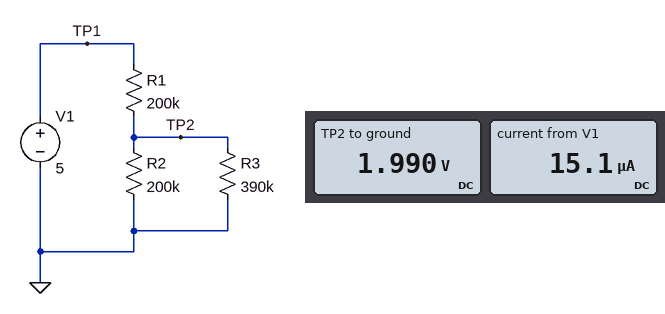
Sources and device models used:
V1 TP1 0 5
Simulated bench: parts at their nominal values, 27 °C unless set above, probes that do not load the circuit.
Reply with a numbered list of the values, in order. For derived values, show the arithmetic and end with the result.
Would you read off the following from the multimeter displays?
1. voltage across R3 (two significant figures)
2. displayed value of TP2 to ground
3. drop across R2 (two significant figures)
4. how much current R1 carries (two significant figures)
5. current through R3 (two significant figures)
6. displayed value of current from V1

1. 1.99 V = 2.0 V
2. 1.990 V
3. 1.99 V = 2.0 V
4. (5 V - 1.99 V) / 200 kΩ = 15 µA
5. (1.99 V) / 390 kΩ = 5.1 µA
6. 15.1 µA
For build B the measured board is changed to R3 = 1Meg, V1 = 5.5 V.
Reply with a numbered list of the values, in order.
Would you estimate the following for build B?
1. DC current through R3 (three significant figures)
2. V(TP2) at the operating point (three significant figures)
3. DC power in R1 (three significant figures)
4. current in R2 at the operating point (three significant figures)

1. 2.50 µA
2. 2.50 V
3. 45.0 µW
4. 12.5 µA
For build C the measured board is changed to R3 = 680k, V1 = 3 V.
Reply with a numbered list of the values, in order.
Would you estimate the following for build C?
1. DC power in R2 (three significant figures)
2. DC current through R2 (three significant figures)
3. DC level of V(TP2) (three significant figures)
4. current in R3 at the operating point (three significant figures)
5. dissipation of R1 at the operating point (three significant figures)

1. 8.55 µW
2. 6.54 µA
3. 1.31 V
4. 1.92 µA
5. 14.3 µW
